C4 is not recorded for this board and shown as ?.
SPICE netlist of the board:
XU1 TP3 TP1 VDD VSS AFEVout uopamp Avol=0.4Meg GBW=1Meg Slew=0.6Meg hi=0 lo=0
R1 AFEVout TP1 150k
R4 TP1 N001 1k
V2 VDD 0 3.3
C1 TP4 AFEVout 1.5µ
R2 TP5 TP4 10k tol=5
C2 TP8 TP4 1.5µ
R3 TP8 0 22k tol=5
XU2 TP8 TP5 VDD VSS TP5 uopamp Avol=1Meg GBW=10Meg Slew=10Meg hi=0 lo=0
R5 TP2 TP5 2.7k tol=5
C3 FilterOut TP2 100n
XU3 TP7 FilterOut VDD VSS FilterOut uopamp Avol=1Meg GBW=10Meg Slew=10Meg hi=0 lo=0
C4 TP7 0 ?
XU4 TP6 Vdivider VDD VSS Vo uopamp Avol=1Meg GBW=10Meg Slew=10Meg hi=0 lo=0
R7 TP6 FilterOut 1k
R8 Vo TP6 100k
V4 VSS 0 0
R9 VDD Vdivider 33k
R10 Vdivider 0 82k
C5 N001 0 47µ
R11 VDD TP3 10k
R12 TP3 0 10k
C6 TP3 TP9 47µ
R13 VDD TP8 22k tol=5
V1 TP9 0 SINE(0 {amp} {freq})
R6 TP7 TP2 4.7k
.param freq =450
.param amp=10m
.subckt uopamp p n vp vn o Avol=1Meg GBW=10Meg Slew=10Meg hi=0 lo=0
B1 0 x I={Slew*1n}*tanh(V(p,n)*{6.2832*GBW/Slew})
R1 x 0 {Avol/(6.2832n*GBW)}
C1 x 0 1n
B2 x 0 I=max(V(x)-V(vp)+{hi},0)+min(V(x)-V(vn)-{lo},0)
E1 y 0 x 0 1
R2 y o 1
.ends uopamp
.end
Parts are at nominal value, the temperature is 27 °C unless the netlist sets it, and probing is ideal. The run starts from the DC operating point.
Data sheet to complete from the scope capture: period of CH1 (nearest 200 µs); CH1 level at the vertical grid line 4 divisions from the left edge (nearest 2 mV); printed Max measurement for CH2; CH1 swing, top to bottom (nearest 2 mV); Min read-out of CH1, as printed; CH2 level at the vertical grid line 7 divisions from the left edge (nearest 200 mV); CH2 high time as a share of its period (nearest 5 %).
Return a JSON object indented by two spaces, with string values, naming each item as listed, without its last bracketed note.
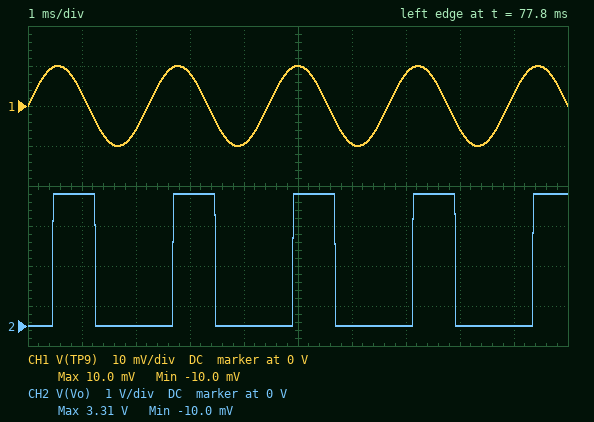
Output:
{
  "period of CH1": "2.2 ms",
  "CH1 level at the vertical grid line 4 divisions from the left edge": "-10 mV",
  "printed Max measurement for CH2": "3.31 V",
  "CH1 swing, top to bottom": "20 mV",
  "Min read-out of CH1, as printed": "-10.0 mV",
  "CH2 level at the vertical grid line 7 divisions from the left edge": "0 V",
  "CH2 high time as a share of its period": "35 %"
}
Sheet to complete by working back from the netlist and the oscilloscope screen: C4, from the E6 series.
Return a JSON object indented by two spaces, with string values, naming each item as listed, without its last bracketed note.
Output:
{
  "C4, from the E6 series": "33 nF"
}
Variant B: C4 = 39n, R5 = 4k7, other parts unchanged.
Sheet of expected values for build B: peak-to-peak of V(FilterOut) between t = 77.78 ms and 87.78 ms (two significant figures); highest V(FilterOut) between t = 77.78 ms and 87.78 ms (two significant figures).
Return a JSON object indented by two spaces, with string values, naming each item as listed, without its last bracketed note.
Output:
{
  "peak-to-peak of V(FilterOut) between t = 77.78 ms and 87.78 ms": "2.8 V",
  "highest V(FilterOut) between t = 77.78 ms and 87.78 ms": "3.0 V"
}
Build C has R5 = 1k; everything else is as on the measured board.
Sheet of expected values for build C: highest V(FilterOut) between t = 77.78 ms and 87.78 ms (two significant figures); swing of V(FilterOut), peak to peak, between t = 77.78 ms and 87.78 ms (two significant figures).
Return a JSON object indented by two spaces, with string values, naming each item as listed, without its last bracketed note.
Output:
{
  "highest V(FilterOut) between t = 77.78 ms and 87.78 ms": "3.1 V",
  "swing of V(FilterOut), peak to peak, between t = 77.78 ms and 87.78 ms": "2.9 V"
}
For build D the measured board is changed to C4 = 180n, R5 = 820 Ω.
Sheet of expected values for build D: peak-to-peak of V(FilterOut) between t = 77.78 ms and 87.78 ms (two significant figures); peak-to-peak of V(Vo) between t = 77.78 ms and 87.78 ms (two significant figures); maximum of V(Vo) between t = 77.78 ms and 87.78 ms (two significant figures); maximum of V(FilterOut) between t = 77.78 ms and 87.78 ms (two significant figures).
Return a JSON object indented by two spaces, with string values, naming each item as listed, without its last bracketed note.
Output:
{
  "peak-to-peak of V(FilterOut) between t = 77.78 ms and 87.78 ms": "1.1 V",
  "peak-to-peak of V(Vo) between t = 77.78 ms and 87.78 ms": "1.6 mV",
  "maximum of V(Vo) between t = 77.78 ms and 87.78 ms": "-8.4 mV",
  "maximum of V(FilterOut) between t = 77.78 ms and 87.78 ms": "2.2 V"
}
